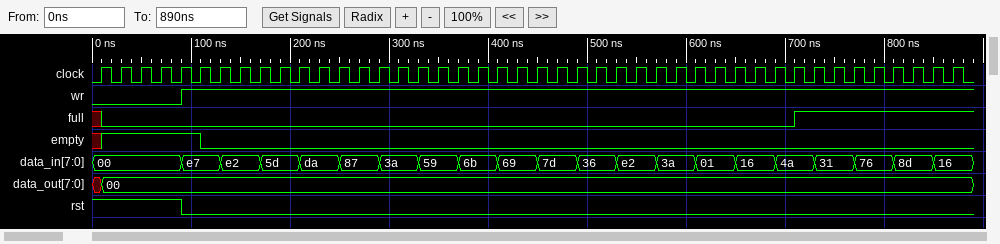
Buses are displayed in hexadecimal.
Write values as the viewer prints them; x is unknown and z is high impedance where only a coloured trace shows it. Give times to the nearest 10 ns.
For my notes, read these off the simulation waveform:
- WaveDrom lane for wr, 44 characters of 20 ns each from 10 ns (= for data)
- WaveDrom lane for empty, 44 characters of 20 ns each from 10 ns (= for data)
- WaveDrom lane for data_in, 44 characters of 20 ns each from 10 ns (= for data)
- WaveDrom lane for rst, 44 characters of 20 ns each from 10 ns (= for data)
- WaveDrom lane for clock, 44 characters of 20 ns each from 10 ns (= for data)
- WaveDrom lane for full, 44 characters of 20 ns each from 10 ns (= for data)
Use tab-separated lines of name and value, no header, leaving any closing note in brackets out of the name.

WaveDrom lane for wr, 44 characters of 20 ns each from 10 ns	{name: 'wr', wave: '0...1.......................................'}
WaveDrom lane for empty, 44 characters of 20 ns each from 10 ns	{name: 'empty', wave: '1....0......................................'}
WaveDrom lane for data_in, 44 characters of 20 ns each from 10 ns	{name: 'data_in', wave: '=...=.=.=.=.=.=.=.=.=.=.=.=.=.=.=.=.=.=.=.=.', data: '00 e7 e2 5d da 87 3a 59 6b 69 7d 36 e2 3a 01 16 4a 31 76 8d 16'}
WaveDrom lane for rst, 44 characters of 20 ns each from 10 ns	{name: 'rst', wave: '1...0.......................................'}
WaveDrom lane for clock, 44 characters of 20 ns each from 10 ns	{name: 'clock', wave: 'p...........................................'}
WaveDrom lane for full, 44 characters of 20 ns each from 10 ns	{name: 'full', wave: '0..................................1........'}
